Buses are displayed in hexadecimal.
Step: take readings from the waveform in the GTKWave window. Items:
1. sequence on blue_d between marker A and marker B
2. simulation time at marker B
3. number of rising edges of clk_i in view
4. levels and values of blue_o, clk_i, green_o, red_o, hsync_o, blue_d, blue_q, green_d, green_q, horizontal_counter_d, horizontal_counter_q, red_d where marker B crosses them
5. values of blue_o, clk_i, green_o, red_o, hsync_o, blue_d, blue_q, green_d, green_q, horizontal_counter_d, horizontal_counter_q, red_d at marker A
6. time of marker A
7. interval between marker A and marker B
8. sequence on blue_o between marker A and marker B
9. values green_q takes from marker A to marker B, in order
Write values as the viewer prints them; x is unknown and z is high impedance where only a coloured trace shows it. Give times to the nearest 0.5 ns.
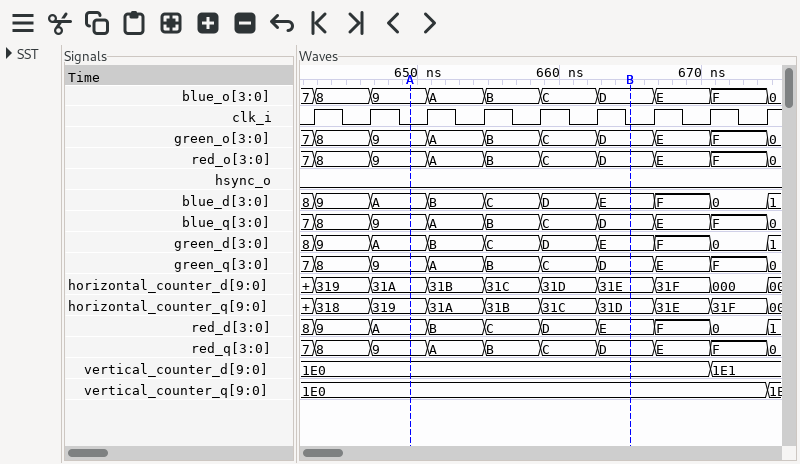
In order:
A, B, C, D, E
665 ns
9
blue_o=D, clk_i=0, green_o=D, red_o=D, hsync_o=0, blue_d=E, blue_q=D, green_d=E, green_q=D, horizontal_counter_d=31E, horizontal_counter_q=31D, red_d=E
blue_o=9, clk_i=0, green_o=9, red_o=9, hsync_o=0, blue_d=A, blue_q=9, green_d=A, green_q=9, horizontal_counter_d=31A, horizontal_counter_q=319, red_d=A
649.5 ns
15.5 ns
9, A, B, C, D
9, A, B, C, D
